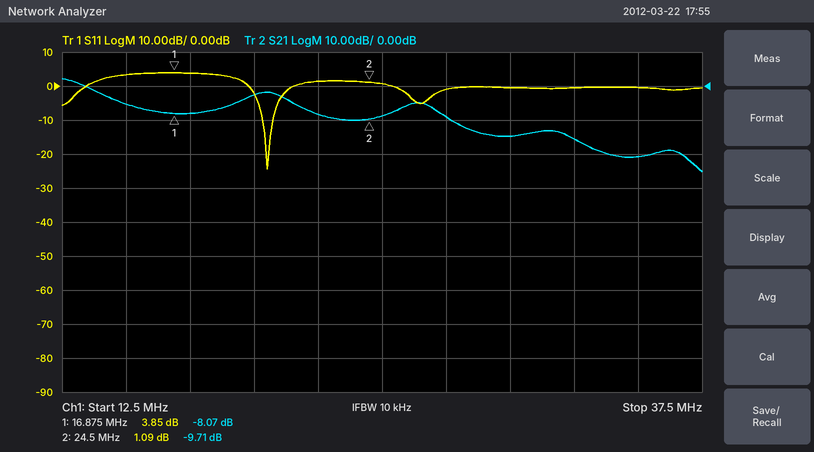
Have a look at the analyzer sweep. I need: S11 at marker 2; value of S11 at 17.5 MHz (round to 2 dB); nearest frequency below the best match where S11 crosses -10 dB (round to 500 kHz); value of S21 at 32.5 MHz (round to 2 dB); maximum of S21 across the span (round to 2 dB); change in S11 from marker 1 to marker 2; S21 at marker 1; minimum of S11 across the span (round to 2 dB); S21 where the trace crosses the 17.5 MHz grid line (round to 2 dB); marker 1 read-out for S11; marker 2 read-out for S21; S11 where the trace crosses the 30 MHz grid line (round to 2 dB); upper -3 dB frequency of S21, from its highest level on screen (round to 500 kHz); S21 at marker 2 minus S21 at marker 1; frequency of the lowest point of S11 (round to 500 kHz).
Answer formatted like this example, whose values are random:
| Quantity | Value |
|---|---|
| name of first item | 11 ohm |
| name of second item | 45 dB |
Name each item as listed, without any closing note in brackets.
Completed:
| Quantity | Value |
|---|---|
| S11 at marker 2 | 1.09 dB |
| value of S11 at 17.5 MHz | 4 dB |
| nearest frequency below the best match where S11 crosses -10 dB | 20.5 MHz |
| value of S21 at 32.5 MHz | -16 dB |
| maximum of S21 across the span | 2 dB |
| change in S11 from marker 1 to marker 2 | -2.76 dB |
| S21 at marker 1 | -8.07 dB |
| minimum of S11 across the span | -24 dB |
| S21 where the trace crosses the 17.5 MHz grid line | -8 dB |
| marker 1 read-out for S11 | 3.85 dB |
| marker 2 read-out for S21 | -9.71 dB |
| S11 where the trace crosses the 30 MHz grid line | 0 dB |
| upper -3 dB frequency of S21, from its highest level on screen | 13.5 MHz |
| S21 at marker 2 minus S21 at marker 1 | -1.64 dB |
| frequency of the lowest point of S11 | 20.5 MHz |
